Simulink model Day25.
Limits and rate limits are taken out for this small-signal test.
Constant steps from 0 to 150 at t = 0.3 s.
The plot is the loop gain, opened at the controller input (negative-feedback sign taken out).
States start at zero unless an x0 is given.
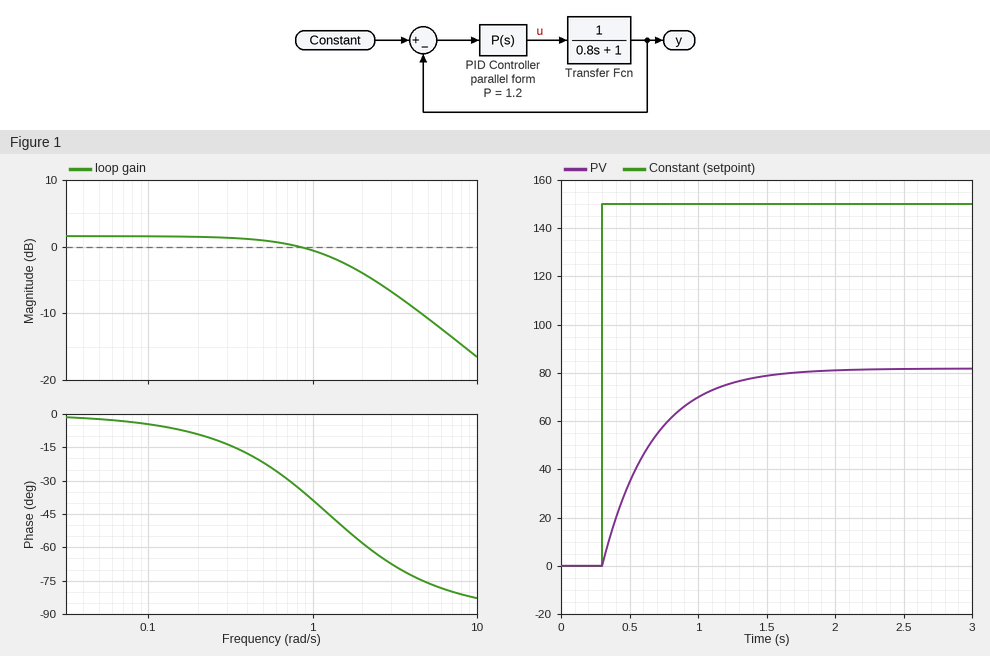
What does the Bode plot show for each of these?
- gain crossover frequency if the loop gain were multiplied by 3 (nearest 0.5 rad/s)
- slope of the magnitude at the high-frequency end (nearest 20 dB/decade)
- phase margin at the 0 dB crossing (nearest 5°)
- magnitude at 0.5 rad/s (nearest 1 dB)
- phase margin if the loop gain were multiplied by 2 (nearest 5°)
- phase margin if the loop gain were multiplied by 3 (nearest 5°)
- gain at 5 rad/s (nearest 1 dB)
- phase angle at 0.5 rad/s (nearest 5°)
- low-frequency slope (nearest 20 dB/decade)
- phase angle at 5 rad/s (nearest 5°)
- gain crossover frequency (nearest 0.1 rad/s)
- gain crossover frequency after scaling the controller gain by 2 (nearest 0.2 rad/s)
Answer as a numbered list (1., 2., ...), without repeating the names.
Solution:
1. 4.5 rad/s
2. -20 dB/decade
3. 145°
4. 1 dB
5. 115°
6. 105°
7. -11 dB
8. -20°
9. 0 dB/decade
10. -75°
11. 0.8 rad/s
12. 2.8 rad/s
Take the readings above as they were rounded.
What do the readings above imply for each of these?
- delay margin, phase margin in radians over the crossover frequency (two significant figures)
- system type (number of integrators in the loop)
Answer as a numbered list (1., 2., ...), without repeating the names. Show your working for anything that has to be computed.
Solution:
1. 145 × π / 180 / 0.8 = 3.2 s
2. 0
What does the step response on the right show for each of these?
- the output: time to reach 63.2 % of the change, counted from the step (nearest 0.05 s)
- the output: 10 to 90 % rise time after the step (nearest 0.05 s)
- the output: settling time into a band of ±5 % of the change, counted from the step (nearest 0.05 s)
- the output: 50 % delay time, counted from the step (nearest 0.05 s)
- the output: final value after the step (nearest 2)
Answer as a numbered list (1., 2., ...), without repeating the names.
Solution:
1. 0.35 s
2. 0.80 s
3. 1.10 s
4. 0.25 s
5. 82
